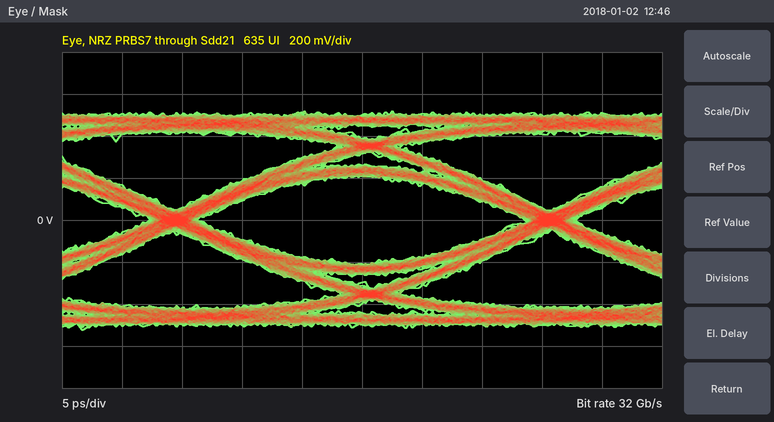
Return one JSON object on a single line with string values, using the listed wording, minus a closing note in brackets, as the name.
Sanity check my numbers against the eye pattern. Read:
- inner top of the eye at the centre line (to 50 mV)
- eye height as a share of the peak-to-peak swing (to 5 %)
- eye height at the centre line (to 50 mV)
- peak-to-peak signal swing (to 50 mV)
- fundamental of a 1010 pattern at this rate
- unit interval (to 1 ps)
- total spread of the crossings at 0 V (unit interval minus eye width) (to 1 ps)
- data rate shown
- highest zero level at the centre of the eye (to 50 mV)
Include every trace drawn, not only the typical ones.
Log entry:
{"inner top of the eye at the centre line": "200 mV", "eye height as a share of the peak-to-peak swing": "40 %", "eye height at the centre line": "400 mV", "peak-to-peak signal swing": "1.05 V", "fundamental of a 1010 pattern at this rate": "16 GHz", "unit interval": "31 ps", "total spread of the crossings at 0 V (unit interval minus eye width)": "4 ps", "data rate shown": "32 Gb/s", "highest zero level at the centre of the eye": "-200 mV"}
